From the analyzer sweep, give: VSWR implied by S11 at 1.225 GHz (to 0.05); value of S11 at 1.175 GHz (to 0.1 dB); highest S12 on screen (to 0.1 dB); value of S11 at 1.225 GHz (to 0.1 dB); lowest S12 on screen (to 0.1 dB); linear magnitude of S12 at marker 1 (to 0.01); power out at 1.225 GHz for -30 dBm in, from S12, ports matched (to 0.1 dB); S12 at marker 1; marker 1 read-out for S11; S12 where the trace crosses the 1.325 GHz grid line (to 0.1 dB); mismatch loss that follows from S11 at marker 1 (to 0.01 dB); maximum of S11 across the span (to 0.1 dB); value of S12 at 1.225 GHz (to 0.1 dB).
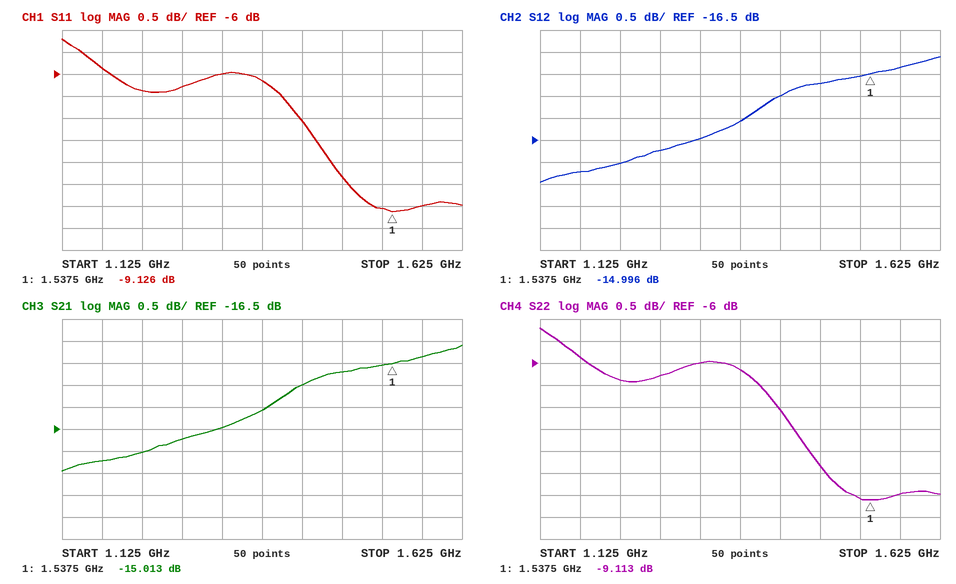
2.85
-5.9 dB
-14.6 dB
-6.4 dB
-17.5 dB
0.18
-47.0 dBm
-14.996 dB
-9.126 dB
-16.5 dB
0.57 dB
-5.2 dB
-17.0 dB
